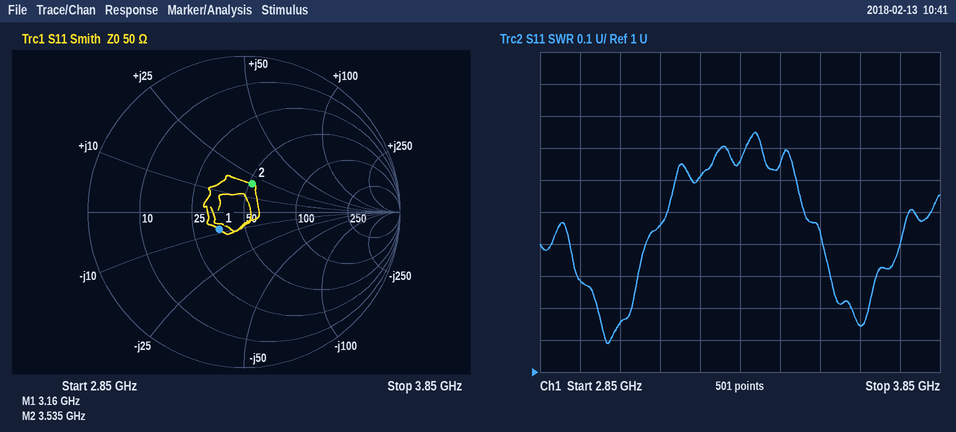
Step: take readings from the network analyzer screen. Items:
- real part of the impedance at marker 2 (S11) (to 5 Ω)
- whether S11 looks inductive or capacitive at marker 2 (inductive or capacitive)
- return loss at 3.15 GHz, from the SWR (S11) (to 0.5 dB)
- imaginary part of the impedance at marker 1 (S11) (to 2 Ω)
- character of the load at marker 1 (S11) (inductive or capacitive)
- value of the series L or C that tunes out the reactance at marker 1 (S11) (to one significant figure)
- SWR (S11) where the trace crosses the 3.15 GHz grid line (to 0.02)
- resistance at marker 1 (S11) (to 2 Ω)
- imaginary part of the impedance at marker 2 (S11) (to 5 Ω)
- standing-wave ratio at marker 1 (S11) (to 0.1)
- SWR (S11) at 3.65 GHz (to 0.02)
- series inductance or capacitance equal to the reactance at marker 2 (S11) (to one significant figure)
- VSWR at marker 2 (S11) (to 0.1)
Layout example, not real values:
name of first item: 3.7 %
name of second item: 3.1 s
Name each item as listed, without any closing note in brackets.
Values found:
real part of the impedance at marker 2 (S11): 50 Ω
whether S11 looks inductive or capacitive at marker 2: inductive
return loss at 3.15 GHz, from the SWR (S11): 14.5 dB
imaginary part of the impedance at marker 1 (S11): -8 Ω
character of the load at marker 1 (S11): capacitive
value of the series L or C that tunes out the reactance at marker 1 (S11): 400 pH
SWR (S11) where the trace crosses the 3.15 GHz grid line: 1.46
resistance at marker 1 (S11): 36 Ω
imaginary part of the impedance at marker 2 (S11): +20 Ω
standing-wave ratio at marker 1 (S11): 1.5
SWR (S11) at 3.65 GHz: 1.14
series inductance or capacitance equal to the reactance at marker 2 (S11): 900 pH
VSWR at marker 2 (S11): 1.5
